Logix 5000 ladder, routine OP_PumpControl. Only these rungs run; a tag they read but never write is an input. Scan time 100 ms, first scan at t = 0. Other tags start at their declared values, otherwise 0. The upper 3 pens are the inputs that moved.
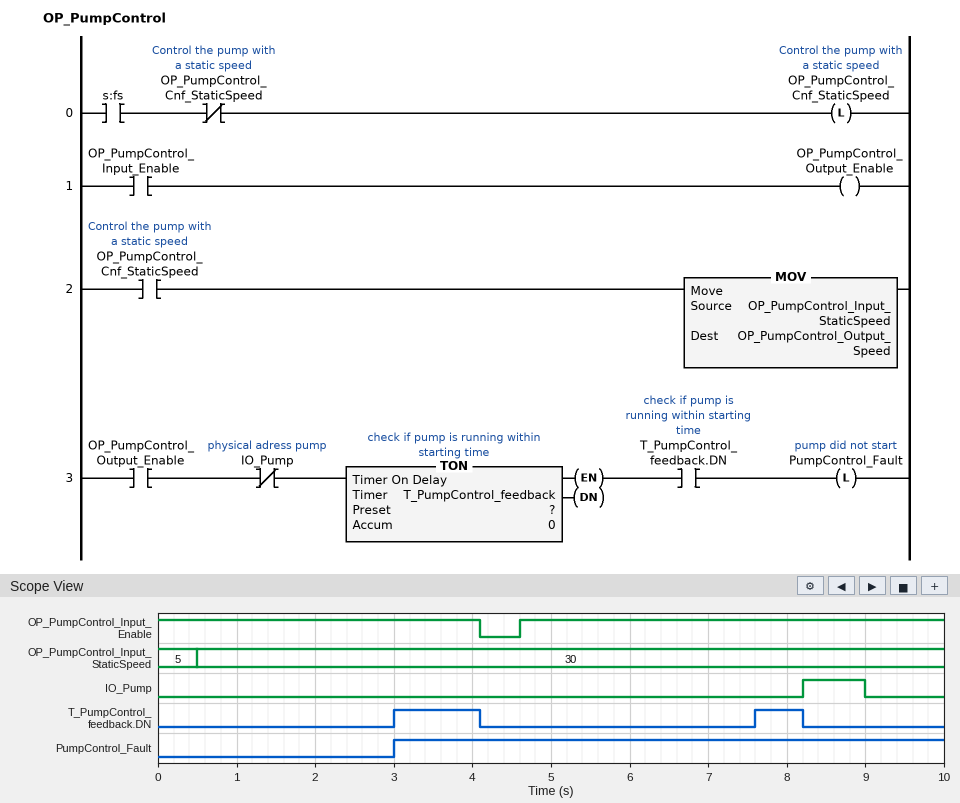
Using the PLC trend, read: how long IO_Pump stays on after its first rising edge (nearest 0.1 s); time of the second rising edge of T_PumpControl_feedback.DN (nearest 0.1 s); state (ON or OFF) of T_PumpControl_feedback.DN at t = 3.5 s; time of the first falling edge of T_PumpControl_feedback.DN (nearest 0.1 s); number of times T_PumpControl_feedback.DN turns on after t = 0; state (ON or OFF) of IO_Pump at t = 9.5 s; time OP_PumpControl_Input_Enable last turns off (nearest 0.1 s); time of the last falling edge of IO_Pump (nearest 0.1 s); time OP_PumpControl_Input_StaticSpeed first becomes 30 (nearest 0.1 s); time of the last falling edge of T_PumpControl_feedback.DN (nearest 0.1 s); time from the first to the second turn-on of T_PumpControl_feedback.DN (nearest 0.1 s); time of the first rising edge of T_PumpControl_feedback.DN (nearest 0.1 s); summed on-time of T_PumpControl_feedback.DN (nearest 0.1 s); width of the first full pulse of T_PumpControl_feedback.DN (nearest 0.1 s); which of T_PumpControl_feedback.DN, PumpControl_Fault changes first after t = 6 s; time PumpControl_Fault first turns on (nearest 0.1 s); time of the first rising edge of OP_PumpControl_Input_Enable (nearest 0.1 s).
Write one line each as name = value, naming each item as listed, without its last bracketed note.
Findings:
how long IO_Pump stays on after its first rising edge = 0.8 s
time of the second rising edge of T_PumpControl_feedback.DN = 7.6 s
state (ON or OFF) of T_PumpControl_feedback.DN at t = 3.5 s = ON
time of the first falling edge of T_PumpControl_feedback.DN = 4.1 s
number of times T_PumpControl_feedback.DN turns on after t = 0 = 2
state (ON or OFF) of IO_Pump at t = 9.5 s = OFF
time OP_PumpControl_Input_Enable last turns off = 4.1 s
time of the last falling edge of IO_Pump = 9.0 s
time OP_PumpControl_Input_StaticSpeed first becomes 30 = 0.5 s
time of the last falling edge of T_PumpControl_feedback.DN = 8.2 s
time from the first to the second turn-on of T_PumpControl_feedback.DN = 4.6 s
time of the first rising edge of T_PumpControl_feedback.DN = 3.0 s
summed on-time of T_PumpControl_feedback.DN = 1.7 s
width of the first full pulse of T_PumpControl_feedback.DN = 1.1 s
which of T_PumpControl_feedback.DN, PumpControl_Fault changes first after t = 6 s = T_PumpControl_feedback.DN
time PumpControl_Fault first turns on = 3.0 s
time of the first rising edge of OP_PumpControl_Input_Enable = 4.6 s
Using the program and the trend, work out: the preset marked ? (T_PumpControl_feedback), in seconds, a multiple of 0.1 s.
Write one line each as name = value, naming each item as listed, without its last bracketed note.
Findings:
the preset marked ? (T_PumpControl_feedback), in seconds, a multiple of 0.1 s = 3.0 s
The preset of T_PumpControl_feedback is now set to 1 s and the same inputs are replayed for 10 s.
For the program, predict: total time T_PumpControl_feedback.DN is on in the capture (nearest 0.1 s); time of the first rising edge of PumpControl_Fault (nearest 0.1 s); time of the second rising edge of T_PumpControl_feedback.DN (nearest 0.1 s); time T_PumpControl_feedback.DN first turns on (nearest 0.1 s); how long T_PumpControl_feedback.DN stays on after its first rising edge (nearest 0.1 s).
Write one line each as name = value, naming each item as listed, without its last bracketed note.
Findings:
total time T_PumpControl_feedback.DN is on in the capture = 5.7 s
time of the first rising edge of PumpControl_Fault = 1.0 s
time of the second rising edge of T_PumpControl_feedback.DN = 5.6 s
time T_PumpControl_feedback.DN first turns on = 1.0 s
how long T_PumpControl_feedback.DN stays on after its first rising edge = 3.1 s
